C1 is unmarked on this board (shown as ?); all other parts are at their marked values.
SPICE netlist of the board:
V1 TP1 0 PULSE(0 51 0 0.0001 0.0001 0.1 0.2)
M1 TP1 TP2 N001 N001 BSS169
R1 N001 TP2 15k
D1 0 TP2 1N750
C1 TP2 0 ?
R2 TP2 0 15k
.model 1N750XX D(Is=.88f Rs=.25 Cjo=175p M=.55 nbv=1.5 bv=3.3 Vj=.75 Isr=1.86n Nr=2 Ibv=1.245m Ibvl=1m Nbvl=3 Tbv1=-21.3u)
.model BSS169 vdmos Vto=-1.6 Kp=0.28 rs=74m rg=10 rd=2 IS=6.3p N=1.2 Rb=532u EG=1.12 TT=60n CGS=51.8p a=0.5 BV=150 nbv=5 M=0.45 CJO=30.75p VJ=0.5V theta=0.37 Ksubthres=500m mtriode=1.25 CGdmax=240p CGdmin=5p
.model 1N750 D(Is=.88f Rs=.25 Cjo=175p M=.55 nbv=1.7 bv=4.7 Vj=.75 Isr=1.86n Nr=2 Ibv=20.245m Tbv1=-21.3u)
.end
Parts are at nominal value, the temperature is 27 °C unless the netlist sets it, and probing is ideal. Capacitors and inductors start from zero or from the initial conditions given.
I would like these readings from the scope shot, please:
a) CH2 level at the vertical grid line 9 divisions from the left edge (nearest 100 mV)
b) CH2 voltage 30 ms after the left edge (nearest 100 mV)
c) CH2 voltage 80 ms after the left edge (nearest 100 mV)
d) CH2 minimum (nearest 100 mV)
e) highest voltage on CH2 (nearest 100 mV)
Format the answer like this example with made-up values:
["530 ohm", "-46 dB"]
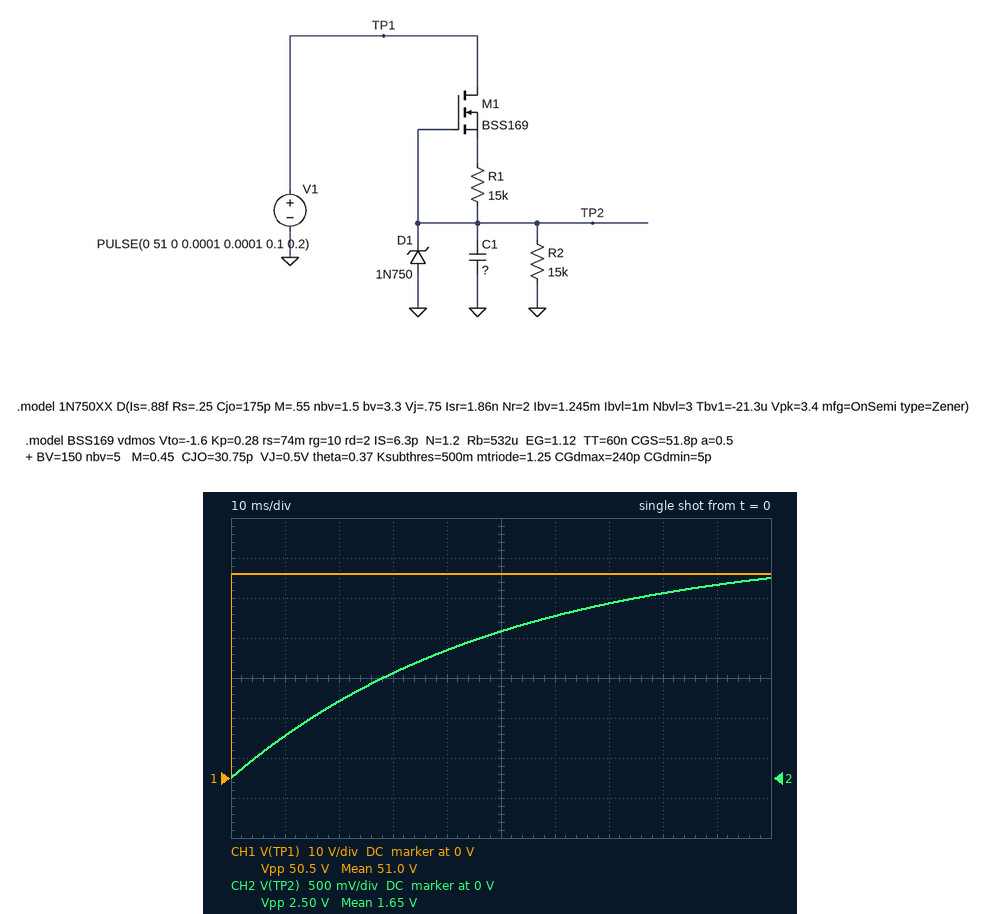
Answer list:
["2.4 V", "1.3 V", "2.3 V", "0 V", "2.5 V"]
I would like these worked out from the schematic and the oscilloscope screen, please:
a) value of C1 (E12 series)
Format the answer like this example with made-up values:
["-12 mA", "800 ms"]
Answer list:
["3.3 µF"]
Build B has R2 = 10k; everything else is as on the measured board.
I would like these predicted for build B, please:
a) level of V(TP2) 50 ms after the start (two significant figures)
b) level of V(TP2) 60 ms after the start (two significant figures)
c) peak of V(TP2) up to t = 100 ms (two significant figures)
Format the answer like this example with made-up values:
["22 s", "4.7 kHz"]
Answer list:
["1.5 V", "1.6 V", "1.8 V"]
